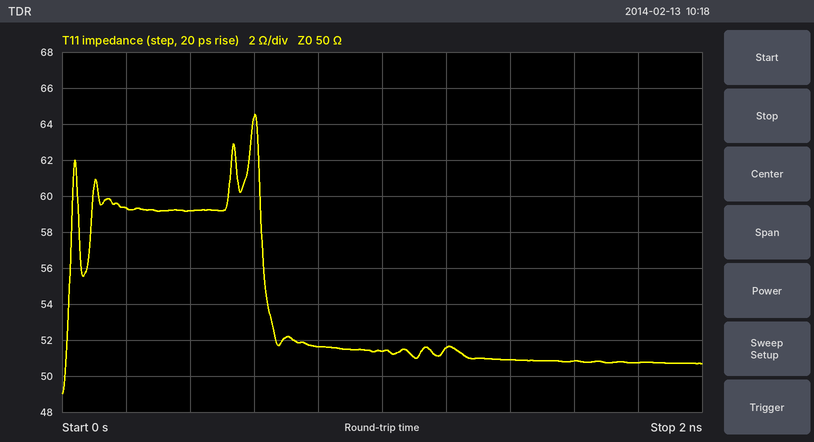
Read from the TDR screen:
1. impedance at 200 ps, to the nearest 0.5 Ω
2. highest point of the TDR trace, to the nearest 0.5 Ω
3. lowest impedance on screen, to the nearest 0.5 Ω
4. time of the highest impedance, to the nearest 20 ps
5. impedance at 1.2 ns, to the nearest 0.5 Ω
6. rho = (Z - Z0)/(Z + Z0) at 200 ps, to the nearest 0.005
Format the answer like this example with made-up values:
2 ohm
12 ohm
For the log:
59.5 Ω
64.5 Ω
49.0 Ω
600 ps
51.5 Ω
+0.085
